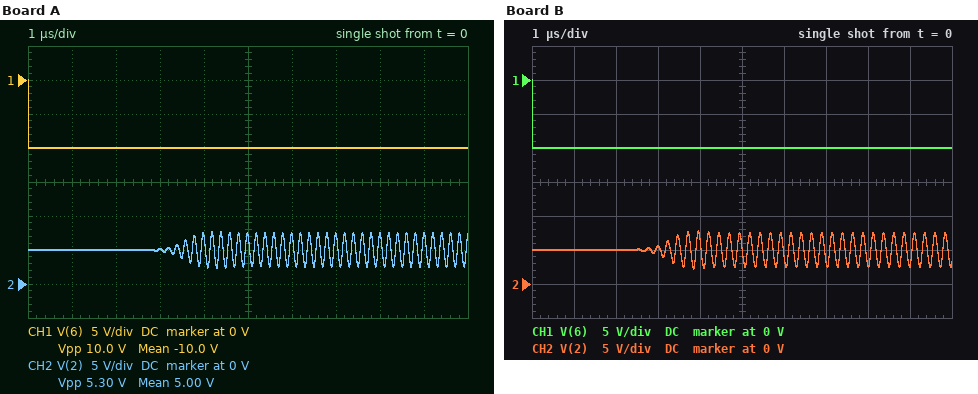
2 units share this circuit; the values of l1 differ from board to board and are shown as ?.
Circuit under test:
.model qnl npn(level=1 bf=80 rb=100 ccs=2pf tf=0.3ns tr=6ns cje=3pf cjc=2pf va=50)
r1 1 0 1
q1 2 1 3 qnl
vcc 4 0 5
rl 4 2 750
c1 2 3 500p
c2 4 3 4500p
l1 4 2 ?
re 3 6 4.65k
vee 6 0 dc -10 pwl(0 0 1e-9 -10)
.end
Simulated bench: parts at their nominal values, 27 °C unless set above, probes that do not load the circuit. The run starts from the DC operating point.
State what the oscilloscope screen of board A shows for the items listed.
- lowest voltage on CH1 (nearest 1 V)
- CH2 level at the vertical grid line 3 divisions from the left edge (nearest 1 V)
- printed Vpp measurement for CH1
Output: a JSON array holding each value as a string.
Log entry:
["-10 V", "5 V", "10.0 V"]
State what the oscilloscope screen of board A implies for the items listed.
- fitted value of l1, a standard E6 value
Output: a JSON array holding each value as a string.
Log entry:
["2.2 µH"]
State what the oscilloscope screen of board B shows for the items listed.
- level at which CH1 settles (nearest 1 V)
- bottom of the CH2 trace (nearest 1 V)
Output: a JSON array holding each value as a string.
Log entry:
["-10 V", "2 V"]
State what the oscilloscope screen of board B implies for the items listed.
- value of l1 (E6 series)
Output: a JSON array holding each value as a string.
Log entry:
["3.3 µH"]
